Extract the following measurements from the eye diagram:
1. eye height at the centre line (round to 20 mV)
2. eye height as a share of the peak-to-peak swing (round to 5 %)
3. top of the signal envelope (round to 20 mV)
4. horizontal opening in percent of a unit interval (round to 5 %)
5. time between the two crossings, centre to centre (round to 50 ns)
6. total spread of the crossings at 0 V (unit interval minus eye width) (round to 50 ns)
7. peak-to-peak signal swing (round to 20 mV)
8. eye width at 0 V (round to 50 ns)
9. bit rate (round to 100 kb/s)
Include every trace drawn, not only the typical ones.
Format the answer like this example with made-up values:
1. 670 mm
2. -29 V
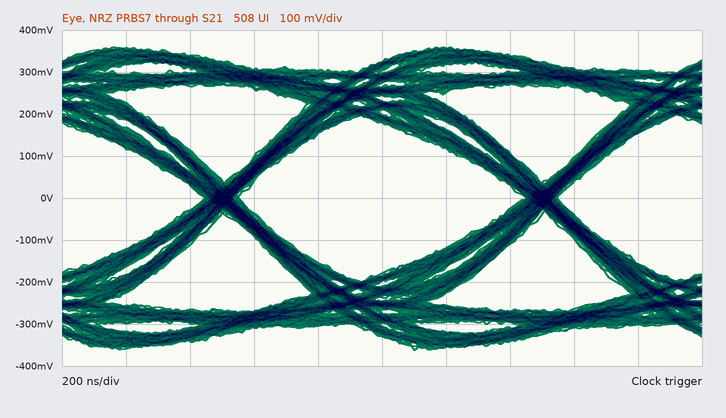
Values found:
1. 360 mV
2. 50 %
3. 360 mV
4. 90 %
5. 1.00 µs
6. 100 ns
7. 720 mV
8. 900 ns
9. 1.0 Mb/s
